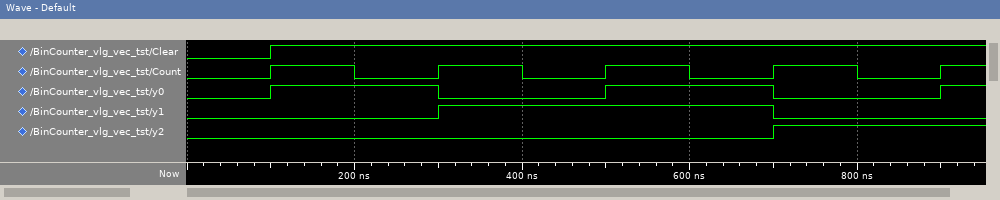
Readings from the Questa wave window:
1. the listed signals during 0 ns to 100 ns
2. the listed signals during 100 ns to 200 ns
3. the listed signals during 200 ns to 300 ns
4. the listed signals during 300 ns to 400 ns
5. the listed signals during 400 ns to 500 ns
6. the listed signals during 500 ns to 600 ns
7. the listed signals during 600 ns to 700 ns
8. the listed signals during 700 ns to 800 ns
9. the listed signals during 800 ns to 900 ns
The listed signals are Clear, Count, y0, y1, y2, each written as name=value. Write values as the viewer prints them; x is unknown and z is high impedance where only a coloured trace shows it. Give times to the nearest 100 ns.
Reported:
Clear=0, Count=0, y0=0, y1=0, y2=0
Clear=1, Count=1, y0=1, y1=0, y2=0
Clear=1, Count=0, y0=1, y1=0, y2=0
Clear=1, Count=1, y0=0, y1=1, y2=0
Clear=1, Count=0, y0=0, y1=1, y2=0
Clear=1, Count=1, y0=1, y1=1, y2=0
Clear=1, Count=0, y0=1, y1=1, y2=0
Clear=1, Count=1, y0=0, y1=0, y2=1
Clear=1, Count=0, y0=0, y1=0, y2=1
